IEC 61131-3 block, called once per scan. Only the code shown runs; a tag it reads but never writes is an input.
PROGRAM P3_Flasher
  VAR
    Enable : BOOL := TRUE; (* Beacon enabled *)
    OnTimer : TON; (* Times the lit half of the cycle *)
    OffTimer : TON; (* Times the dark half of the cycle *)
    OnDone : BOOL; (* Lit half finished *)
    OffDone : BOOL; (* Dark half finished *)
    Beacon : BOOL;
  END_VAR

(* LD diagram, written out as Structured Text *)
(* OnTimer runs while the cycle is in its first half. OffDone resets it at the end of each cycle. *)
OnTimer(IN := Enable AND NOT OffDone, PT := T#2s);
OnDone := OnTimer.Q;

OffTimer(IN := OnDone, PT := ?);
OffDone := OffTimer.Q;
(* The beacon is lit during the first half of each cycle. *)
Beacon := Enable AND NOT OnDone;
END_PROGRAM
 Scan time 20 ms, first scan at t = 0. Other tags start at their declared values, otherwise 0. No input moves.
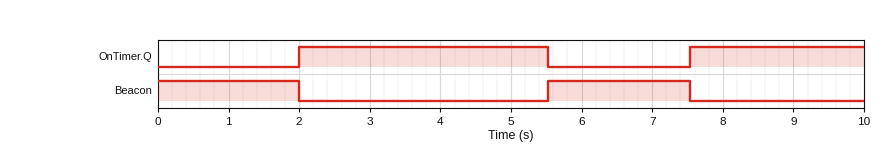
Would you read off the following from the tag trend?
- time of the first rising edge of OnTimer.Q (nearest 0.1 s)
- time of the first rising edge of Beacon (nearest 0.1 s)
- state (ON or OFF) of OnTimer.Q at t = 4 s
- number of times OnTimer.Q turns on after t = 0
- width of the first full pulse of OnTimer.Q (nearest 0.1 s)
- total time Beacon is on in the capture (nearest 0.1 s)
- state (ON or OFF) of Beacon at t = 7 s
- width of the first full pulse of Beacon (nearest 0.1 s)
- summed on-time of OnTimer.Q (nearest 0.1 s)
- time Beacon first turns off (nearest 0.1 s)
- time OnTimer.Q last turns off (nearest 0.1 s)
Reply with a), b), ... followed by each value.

a) 2.0 s
b) 5.5 s
c) ON
d) 2
e) 3.5 s
f) 4.0 s
g) ON
h) 2.0 s
i) 6.0 s
j) 2.0 s
k) 5.5 s
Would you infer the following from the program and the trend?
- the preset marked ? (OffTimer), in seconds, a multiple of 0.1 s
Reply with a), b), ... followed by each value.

a) 3.5 s
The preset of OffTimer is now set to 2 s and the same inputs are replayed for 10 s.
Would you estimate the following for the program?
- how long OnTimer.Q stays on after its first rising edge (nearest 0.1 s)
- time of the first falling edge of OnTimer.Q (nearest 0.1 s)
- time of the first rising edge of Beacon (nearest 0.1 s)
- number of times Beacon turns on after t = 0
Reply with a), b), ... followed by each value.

a) 2.0 s
b) 4.0 s
c) 4.0 s
d) 2
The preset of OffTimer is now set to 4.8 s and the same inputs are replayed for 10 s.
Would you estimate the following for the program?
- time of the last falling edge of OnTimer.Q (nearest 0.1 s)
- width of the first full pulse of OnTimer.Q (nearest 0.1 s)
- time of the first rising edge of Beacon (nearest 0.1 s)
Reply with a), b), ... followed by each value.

a) 6.8 s
b) 4.8 s
c) 6.8 s
